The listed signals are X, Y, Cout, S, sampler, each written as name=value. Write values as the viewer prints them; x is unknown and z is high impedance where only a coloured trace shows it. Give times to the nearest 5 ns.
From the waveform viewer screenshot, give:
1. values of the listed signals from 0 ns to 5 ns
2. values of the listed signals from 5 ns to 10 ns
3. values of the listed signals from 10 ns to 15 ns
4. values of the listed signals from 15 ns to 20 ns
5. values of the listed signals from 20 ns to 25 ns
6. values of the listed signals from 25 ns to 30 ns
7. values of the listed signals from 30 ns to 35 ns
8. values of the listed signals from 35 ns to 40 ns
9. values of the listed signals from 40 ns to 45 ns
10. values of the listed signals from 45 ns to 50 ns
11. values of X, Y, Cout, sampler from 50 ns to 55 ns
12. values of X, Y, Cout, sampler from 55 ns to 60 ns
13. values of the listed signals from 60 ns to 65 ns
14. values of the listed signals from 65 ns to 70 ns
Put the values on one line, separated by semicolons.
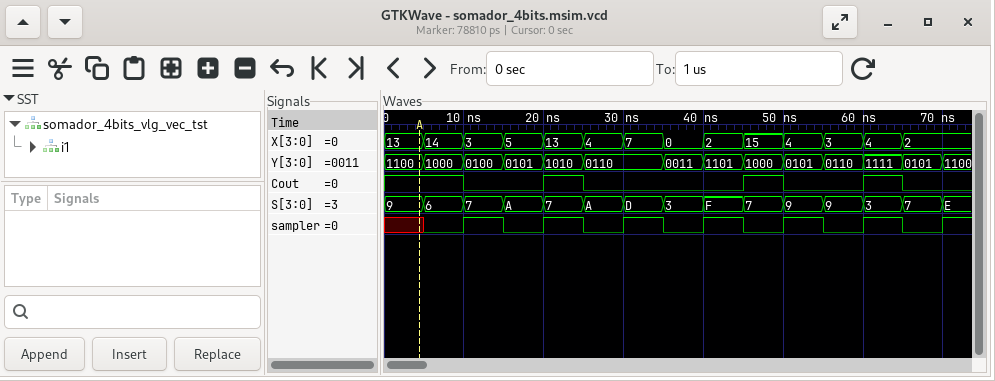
X=13, Y=1100, Cout=1, S=9, sampler=x; X=14, Y=1000, Cout=1, S=6, sampler=0; X=3, Y=0100, Cout=0, S=7, sampler=1; X=5, Y=0101, Cout=0, S=A, sampler=0; X=13, Y=1010, Cout=1, S=7, sampler=1; X=4, Y=0110, Cout=0, S=A, sampler=0; X=7, Y=0110, Cout=0, S=D, sampler=1; X=0, Y=0011, Cout=0, S=3, sampler=0; X=2, Y=1101, Cout=0, S=F, sampler=1; X=15, Y=1000, Cout=1, S=7, sampler=0; X=4, Y=0101, Cout=0, sampler=1; X=3, Y=0110, Cout=0, sampler=0; X=4, Y=1111, Cout=1, S=3, sampler=1; X=2, Y=0101, Cout=0, S=7, sampler=0
